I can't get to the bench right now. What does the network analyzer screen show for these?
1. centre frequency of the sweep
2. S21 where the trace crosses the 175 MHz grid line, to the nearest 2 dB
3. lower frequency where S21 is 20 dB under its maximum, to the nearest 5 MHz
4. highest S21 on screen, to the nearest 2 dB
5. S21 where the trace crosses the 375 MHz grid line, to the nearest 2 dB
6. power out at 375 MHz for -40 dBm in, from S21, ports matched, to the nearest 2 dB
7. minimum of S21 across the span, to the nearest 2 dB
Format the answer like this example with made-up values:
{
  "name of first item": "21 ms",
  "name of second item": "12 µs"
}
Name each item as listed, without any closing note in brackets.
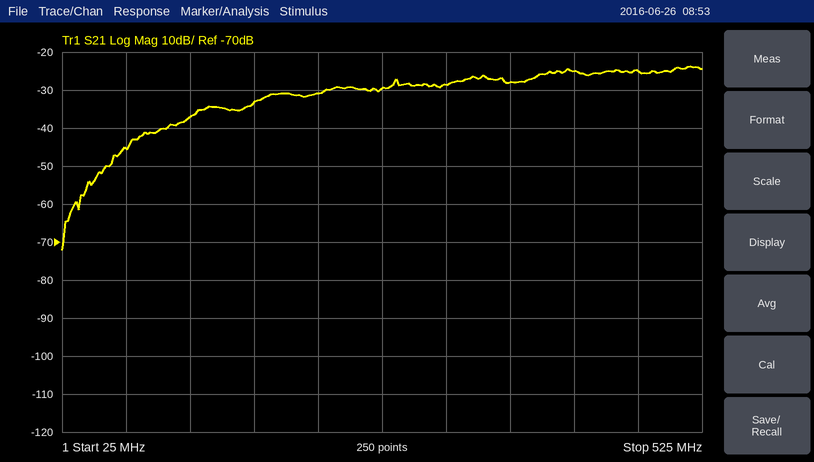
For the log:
{
  "centre frequency of the sweep": "275 MHz",
  "S21 where the trace crosses the 175 MHz grid line, to the nearest 2 dB": "-34 dB",
  "lower frequency where S21 is 20 dB under its maximum, to the nearest 5 MHz": "80 MHz",
  "highest S21 on screen, to the nearest 2 dB": "-24 dB",
  "S21 where the trace crosses the 375 MHz grid line, to the nearest 2 dB": "-28 dB",
  "power out at 375 MHz for -40 dBm in, from S21, ports matched, to the nearest 2 dB": "-68 dBm",
  "minimum of S21 across the span, to the nearest 2 dB": "-72 dB"
}
